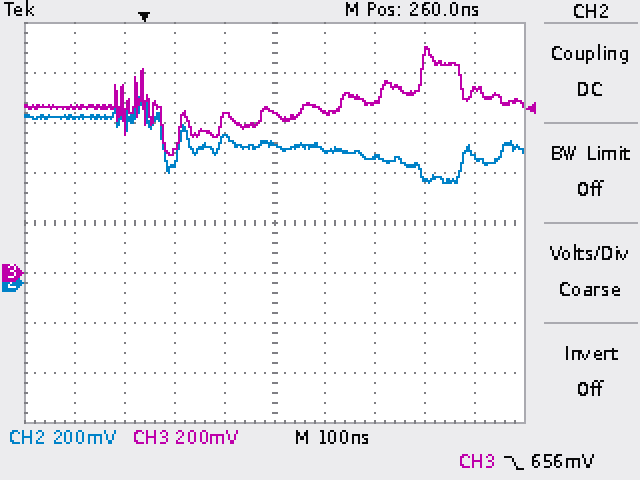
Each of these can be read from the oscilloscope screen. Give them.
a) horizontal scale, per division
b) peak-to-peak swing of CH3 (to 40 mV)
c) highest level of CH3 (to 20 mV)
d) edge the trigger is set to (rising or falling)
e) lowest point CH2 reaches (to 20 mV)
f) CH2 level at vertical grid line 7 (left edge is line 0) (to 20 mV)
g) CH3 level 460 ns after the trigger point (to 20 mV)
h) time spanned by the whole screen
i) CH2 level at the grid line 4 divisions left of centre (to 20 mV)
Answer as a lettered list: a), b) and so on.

a) 100 ns
b) 440 mV
c) 900 mV
d) falling
e) 400 mV
f) 500 mV
g) 680 mV
h) 1 µs
i) 660 mV
